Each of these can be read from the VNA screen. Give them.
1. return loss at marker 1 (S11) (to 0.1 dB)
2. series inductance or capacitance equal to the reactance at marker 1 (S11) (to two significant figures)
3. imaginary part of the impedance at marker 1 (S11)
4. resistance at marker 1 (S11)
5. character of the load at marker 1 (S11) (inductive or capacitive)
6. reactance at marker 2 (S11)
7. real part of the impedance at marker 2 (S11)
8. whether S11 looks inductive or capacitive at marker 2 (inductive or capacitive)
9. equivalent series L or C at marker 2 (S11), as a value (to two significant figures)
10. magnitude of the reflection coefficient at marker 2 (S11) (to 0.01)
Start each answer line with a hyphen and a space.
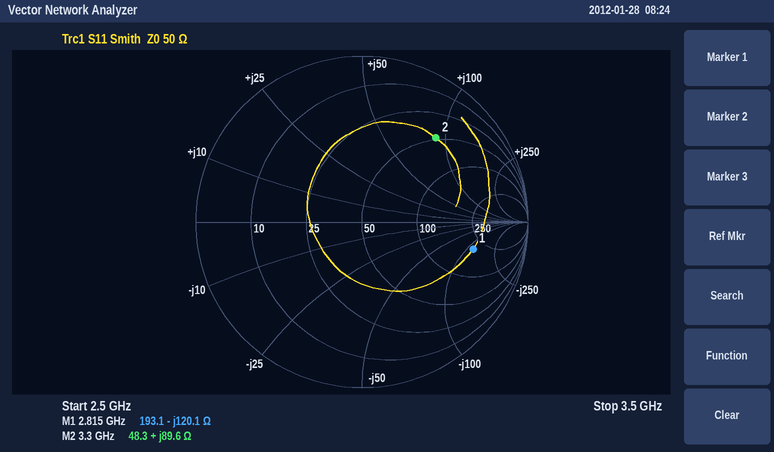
- 3.2 dB
- 470 fF
- -120.1 Ω
- 193.1 Ω
- capacitive
- +89.6 Ω
- 48.3 Ω
- inductive
- 4.3 nH
- 0.67
